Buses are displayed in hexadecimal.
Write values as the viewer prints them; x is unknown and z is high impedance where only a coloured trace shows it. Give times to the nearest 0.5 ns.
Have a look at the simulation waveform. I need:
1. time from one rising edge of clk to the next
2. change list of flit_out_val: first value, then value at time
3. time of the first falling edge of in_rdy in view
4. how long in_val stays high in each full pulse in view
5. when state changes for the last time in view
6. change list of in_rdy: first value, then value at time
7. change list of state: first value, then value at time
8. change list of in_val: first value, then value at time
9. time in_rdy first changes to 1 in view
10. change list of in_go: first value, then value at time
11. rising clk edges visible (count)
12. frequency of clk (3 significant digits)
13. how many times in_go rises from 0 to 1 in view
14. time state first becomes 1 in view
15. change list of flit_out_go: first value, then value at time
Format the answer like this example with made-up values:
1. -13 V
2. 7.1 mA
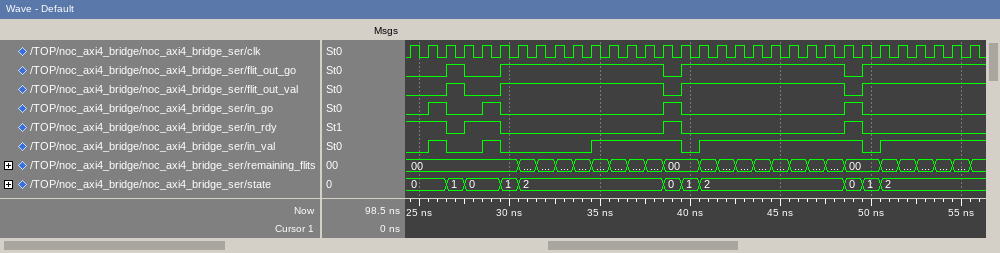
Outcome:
1. 1 ns
2. 0, 1 at 26.5 ns, 0 at 27.5 ns, 1 at 29.5 ns, 0 at 38.5 ns, 1 at 39.5 ns, 0 at 48.5 ns, 1 at 49.5 ns
3. 26.5 ns
4. 1 ns, 1 ns, 5 ns, 9 ns
5. 50.5 ns
6. 1, 0 at 26.5 ns, 1 at 27.5 ns, 0 at 29.5 ns, 1 at 38.5 ns, 0 at 39.5 ns, 1 at 48.5 ns, 0 at 49.5 ns
7. 0, 1 at 26.5 ns, 0 at 27.5 ns, 1 at 29.5 ns, 2 at 30.5 ns, 0 at 38.5 ns, 1 at 39.5 ns, 2 at 40.5 ns, 0 at 48.5 ns, 1 at 49.5 ns, 2 at 50.5 ns
8. 0, 1 at 25.5 ns, 0 at 26.5 ns, 1 at 28.5 ns, 0 at 29.5 ns, 1 at 34.5 ns, 0 at 39.5 ns, 1 at 40.5 ns, 0 at 49.5 ns, 1 at 50.5 ns
9. 27.5 ns
10. 0, 1 at 25.5 ns, 0 at 26.5 ns, 1 at 28.5 ns, 0 at 29.5 ns, 1 at 38.5 ns, 0 at 39.5 ns, 1 at 48.5 ns, 0 at 49.5 ns
11. 32
12. 1.00 GHz
13. 4
14. 26.5 ns
15. 0, 1 at 26.5 ns, 0 at 27.5 ns, 1 at 29.5 ns, 0 at 38.5 ns, 1 at 39.5 ns, 0 at 48.5 ns, 1 at 49.5 ns
